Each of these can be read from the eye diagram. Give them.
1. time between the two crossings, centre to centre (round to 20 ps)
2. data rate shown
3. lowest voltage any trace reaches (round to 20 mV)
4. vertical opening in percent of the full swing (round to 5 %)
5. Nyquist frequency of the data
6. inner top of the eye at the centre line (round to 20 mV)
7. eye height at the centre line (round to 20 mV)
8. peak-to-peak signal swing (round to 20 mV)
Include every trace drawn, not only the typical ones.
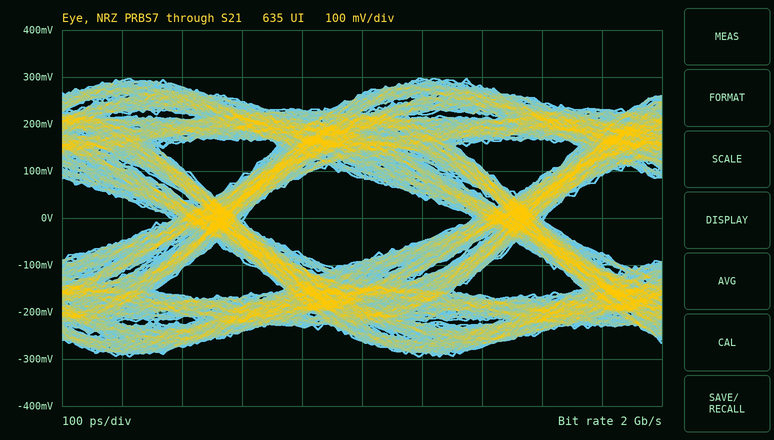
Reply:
500 ps
2 Gb/s
-300 mV
30 %
1 GHz
80 mV
180 mV
600 mV
